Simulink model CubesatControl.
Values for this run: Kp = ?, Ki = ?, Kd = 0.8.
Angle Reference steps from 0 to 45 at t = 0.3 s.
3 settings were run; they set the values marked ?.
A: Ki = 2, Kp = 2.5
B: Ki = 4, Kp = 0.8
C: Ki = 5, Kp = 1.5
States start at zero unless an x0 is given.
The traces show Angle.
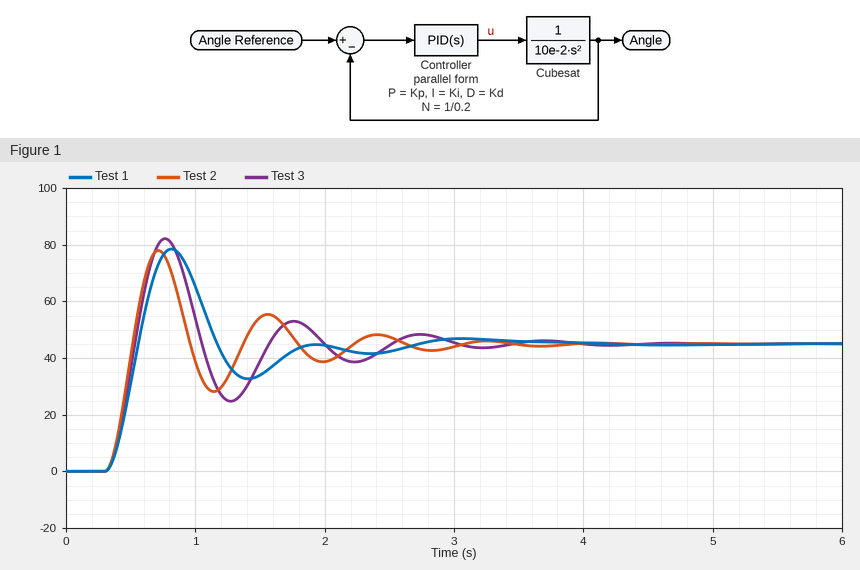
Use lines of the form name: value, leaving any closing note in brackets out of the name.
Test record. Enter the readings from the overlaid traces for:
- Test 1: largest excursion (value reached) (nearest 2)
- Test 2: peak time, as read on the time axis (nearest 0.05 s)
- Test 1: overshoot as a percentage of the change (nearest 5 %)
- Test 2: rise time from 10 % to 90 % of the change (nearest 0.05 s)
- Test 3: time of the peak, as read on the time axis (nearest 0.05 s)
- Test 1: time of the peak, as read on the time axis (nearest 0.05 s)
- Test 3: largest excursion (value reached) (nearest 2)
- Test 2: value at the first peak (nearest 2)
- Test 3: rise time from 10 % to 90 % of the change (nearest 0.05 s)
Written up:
Test 1: largest excursion (value reached): 78
Test 2: peak time, as read on the time axis: 0.70 s
Test 1: overshoot as a percentage of the change: 75 %
Test 2: rise time from 10 % to 90 % of the change: 0.15 s
Test 3: time of the peak, as read on the time axis: 0.75 s
Test 1: time of the peak, as read on the time axis: 0.80 s
Test 3: largest excursion (value reached): 82
Test 2: value at the first peak: 78
Test 3: rise time from 10 % to 90 % of the change: 0.15 s
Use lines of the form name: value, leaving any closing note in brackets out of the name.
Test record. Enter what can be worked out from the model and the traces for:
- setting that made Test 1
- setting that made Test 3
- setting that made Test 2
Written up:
setting that made Test 1: B
setting that made Test 3: C
setting that made Test 2: A
